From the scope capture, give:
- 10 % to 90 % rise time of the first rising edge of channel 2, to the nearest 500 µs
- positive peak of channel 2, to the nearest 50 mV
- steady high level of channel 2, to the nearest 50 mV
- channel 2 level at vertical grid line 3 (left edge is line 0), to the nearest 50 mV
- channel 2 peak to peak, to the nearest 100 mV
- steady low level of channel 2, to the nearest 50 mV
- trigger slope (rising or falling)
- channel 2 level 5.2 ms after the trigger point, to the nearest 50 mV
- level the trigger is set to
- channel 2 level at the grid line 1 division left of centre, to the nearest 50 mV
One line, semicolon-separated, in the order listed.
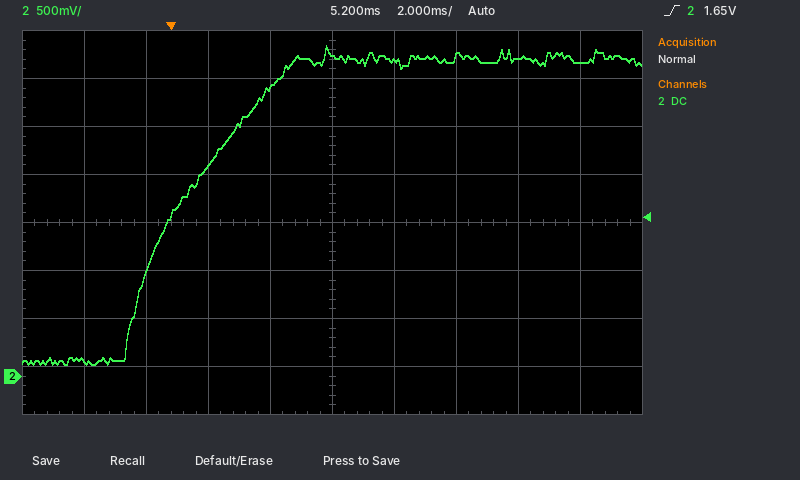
4.5 ms; 3.45 V; 3.30 V; 2.20 V; 3.30 V; 150 mV; rising; 3.35 V; 1.65 V; 3.00 V
